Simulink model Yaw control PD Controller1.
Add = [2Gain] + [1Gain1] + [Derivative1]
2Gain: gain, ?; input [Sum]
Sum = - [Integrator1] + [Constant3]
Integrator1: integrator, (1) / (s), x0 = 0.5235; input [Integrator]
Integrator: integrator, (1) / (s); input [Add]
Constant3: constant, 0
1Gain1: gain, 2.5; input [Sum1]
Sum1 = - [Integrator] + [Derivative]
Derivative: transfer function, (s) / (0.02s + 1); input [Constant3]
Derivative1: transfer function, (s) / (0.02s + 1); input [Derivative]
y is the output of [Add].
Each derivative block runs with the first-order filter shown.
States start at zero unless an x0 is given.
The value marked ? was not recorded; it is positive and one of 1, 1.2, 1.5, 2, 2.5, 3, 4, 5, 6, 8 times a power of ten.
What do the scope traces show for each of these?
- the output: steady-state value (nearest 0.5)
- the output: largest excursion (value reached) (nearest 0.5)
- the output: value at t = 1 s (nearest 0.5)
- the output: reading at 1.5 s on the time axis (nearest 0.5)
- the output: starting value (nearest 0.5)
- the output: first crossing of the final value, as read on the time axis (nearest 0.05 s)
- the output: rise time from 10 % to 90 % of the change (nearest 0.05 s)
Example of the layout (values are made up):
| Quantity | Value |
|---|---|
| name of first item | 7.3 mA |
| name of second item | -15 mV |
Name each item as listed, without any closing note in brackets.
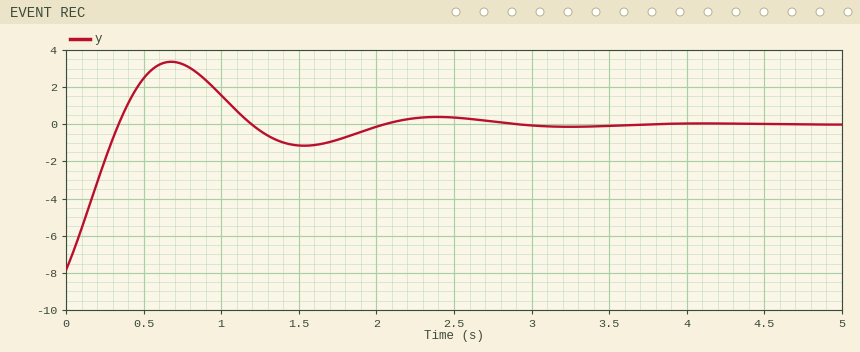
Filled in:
| Quantity | Value |
|---|---|
| the output: steady-state value | 0.0 |
| the output: largest excursion (value reached) | 3.5 |
| the output: value at t = 1 s | 1.5 |
| the output: reading at 1.5 s on the time axis | -1.0 |
| the output: starting value | -8.0 |
| the output: first crossing of the final value, as read on the time axis | 0.35 s |
| the output: rise time from 10 % to 90 % of the change | 0.25 s |
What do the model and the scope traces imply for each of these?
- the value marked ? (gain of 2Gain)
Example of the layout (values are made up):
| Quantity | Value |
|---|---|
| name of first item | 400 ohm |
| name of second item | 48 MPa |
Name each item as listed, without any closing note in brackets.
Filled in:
| Quantity | Value |
|---|---|
| the value marked ? | 15 |
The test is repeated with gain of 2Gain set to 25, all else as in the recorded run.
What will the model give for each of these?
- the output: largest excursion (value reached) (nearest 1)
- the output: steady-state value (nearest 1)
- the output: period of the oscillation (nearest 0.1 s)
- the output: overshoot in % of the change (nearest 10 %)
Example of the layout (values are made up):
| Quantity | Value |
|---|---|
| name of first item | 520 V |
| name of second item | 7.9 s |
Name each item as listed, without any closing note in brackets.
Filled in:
| Quantity | Value |
|---|---|
| the output: largest excursion (value reached) | 7 |
| the output: steady-state value | 0 |
| the output: period of the oscillation | 1.3 s |
| the output: overshoot in % of the change | 50 % |
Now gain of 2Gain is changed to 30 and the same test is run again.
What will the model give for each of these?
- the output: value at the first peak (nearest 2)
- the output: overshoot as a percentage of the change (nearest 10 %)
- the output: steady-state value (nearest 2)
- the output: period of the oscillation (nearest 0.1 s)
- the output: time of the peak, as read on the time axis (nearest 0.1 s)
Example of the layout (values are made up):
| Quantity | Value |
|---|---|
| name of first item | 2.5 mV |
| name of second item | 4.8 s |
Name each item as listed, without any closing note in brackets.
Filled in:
| Quantity | Value |
|---|---|
| the output: value at the first peak | 8 |
| the output: overshoot as a percentage of the change | 50 % |
| the output: steady-state value | 0 |
| the output: period of the oscillation | 1.2 s |
| the output: time of the peak, as read on the time axis | 0.5 s |
